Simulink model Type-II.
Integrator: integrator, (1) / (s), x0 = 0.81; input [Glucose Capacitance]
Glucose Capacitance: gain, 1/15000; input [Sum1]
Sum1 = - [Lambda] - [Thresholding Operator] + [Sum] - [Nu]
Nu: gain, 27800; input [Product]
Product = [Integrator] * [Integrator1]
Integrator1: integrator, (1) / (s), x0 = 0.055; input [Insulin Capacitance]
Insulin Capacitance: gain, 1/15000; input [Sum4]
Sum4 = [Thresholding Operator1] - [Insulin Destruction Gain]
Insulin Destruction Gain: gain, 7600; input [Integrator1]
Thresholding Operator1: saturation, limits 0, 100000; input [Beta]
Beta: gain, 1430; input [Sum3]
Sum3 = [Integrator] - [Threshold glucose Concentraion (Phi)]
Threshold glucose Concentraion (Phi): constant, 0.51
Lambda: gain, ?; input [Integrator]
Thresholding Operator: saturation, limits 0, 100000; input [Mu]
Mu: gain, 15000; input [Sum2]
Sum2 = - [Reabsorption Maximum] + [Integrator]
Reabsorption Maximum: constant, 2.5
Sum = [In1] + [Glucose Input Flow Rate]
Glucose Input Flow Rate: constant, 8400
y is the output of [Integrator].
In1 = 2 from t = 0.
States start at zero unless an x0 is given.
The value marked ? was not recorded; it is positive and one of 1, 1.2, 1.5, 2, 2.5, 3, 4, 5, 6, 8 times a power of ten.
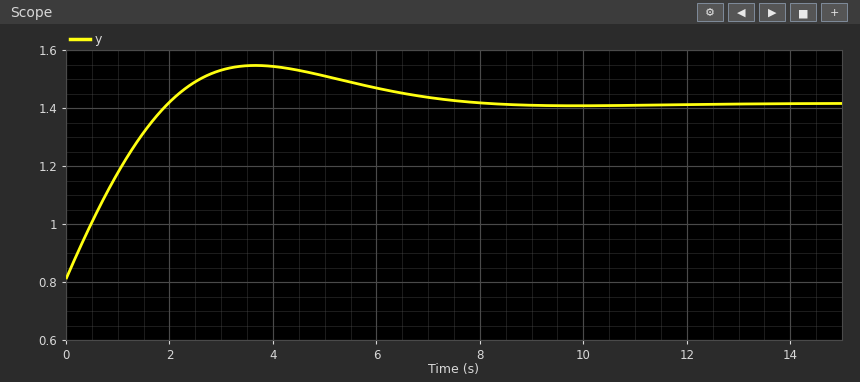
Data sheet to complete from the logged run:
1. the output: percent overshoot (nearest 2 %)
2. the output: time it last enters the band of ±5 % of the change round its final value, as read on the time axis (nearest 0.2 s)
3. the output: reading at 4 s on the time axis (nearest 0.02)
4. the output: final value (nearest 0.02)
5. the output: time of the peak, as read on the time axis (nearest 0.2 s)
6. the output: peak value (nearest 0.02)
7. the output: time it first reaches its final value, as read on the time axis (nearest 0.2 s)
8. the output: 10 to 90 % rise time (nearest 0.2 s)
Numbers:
22 %
6.6 s
1.54
1.42
3.6 s
1.54
2.0 s
1.6 s
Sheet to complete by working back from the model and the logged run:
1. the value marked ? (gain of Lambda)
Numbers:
1200
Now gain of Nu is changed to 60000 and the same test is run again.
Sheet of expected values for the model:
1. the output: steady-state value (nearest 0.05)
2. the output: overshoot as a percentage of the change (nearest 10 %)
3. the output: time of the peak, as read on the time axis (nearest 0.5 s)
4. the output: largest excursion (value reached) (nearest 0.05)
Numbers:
1.10
40 %
2.5 s
1.20
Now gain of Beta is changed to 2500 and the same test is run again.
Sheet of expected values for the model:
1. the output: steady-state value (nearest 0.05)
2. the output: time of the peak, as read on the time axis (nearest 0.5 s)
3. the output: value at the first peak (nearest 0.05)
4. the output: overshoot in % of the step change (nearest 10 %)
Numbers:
1.15
2.5 s
1.35
50 %
